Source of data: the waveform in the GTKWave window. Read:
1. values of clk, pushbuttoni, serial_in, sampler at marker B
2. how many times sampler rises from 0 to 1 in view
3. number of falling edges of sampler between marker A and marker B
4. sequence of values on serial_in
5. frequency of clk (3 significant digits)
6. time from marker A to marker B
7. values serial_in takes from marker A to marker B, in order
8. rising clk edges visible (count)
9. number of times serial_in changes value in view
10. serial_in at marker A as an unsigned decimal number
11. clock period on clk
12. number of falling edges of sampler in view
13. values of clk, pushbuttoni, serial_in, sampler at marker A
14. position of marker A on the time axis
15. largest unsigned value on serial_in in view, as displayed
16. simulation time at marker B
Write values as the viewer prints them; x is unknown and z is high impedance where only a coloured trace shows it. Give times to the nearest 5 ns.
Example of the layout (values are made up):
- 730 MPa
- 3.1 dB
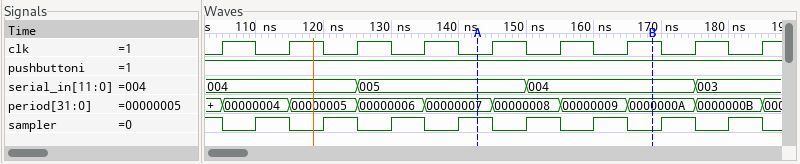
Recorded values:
- clk=1, pushbuttoni=1, serial_in=004, sampler=0
- 8
- 3
- 004, 005, 004, 003
- 100 MHz
- 25 ns
- 005, 004
- 9
- 3
- 5
- 10 ns
- 9
- clk=0, pushbuttoni=1, serial_in=005, sampler=1
- 145 ns
- 005
- 170 ns
